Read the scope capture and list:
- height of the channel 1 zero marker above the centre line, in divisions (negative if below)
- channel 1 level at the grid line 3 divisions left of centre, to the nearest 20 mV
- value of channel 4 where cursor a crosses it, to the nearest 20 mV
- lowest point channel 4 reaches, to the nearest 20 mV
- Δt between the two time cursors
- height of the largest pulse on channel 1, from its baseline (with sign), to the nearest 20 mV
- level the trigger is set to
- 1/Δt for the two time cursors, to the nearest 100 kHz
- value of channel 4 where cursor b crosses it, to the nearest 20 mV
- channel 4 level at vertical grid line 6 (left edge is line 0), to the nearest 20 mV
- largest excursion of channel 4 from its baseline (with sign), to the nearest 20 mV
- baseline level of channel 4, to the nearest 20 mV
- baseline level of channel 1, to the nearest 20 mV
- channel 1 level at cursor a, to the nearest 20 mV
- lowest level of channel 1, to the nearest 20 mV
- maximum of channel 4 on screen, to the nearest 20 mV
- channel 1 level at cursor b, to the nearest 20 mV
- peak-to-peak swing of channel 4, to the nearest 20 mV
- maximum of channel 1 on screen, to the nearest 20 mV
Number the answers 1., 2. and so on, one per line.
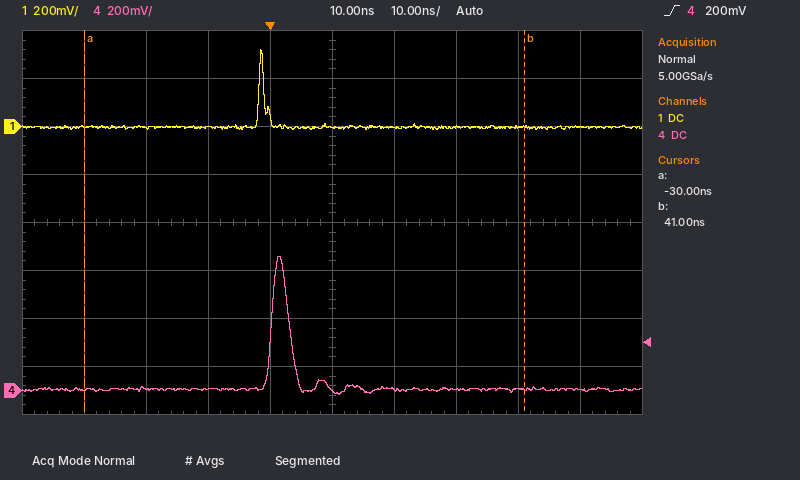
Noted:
1. +2.0 div
2. 0 mV
3. 0 mV
4. -20 mV
5. 71 ns
6. +320 mV
7. 200 mV
8. 14.1 MHz
9. 0 mV
10. 0 mV
11. +560 mV
12. 0 mV
13. 0 mV
14. 0 mV
15. -20 mV
16. 560 mV
17. 0 mV
18. 580 mV
19. 320 mV
